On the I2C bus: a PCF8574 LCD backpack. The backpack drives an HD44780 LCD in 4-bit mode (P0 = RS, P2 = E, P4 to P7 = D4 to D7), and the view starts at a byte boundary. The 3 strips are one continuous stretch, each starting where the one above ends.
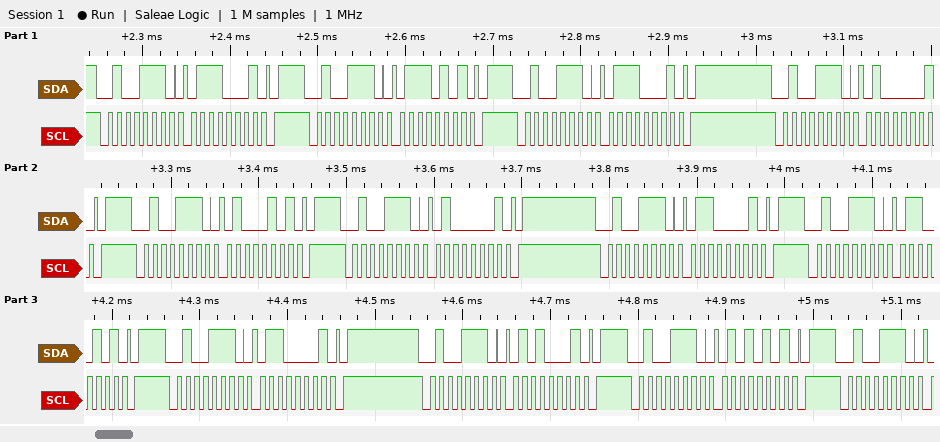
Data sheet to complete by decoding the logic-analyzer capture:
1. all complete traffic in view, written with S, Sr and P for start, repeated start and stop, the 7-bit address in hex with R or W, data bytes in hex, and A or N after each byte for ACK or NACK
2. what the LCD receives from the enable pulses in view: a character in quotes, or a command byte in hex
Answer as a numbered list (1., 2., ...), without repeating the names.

1. S 27W A 71 A P S 27W A 75 A P S 27W A 71 A P S 27W A 41 A P S 27W A 45 A P S 27W A 41 A P S 27W A 61 A P S 27W A 65 A P S 27W A 61 A P S 27W A 51 A P S 27W A 55 A P S 27W A
2. 't'
